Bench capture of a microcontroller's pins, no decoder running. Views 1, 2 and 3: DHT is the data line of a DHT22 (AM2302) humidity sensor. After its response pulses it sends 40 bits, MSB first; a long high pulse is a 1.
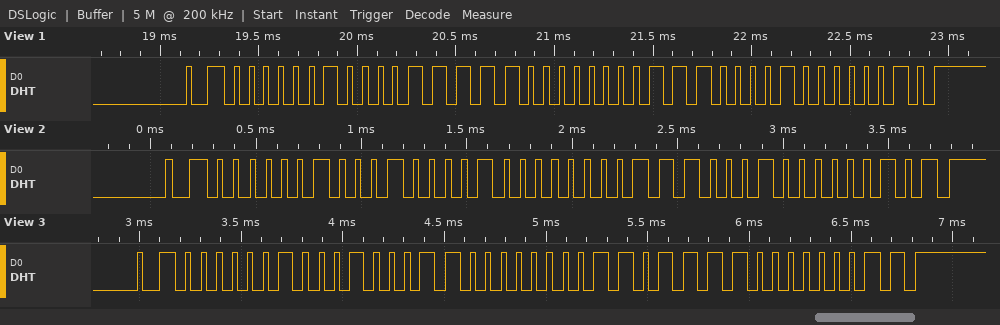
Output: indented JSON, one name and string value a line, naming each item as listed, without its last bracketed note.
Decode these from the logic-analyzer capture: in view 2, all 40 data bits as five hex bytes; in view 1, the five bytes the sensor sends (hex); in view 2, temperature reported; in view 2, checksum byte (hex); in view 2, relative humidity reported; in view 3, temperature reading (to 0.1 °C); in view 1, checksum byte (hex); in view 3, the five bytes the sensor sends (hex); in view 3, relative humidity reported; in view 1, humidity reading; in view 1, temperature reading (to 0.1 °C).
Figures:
{
  "in view 2, all 40 data bits as five hex bytes": "02 21 00 E2 05",
  "in view 1, the five bytes the sensor sends": "02 1F 00 E1 02",
  "in view 2, temperature reported": "22.6 °C",
  "in view 2, checksum byte": "0x05",
  "in view 2, relative humidity reported": "54.5 %",
  "in view 3, temperature reading": "22.2 °C",
  "in view 1, checksum byte": "0x02",
  "in view 3, the five bytes the sensor sends": "02 23 00 DE 03",
  "in view 3, relative humidity reported": "54.7 %",
  "in view 1, humidity reading": "54.3 %",
  "in view 1, temperature reading": "22.5 °C"
}
